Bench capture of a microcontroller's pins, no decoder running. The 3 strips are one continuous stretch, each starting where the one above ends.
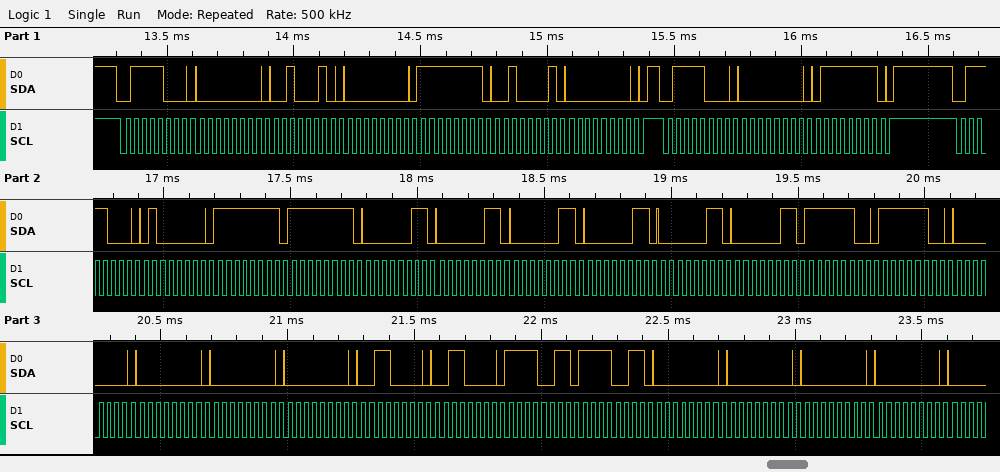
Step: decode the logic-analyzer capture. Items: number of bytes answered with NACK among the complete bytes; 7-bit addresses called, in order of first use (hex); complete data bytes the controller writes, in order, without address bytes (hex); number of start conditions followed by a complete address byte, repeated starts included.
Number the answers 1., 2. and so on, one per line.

1. 0
2. 0x3C
3. 00 22 00 FF 21 00 00 7F 40 FF FF 03 03 03 03 03 03 FC FC 00 00 00 00 30 30 F3 F3 00 00 00 00
4. 3
